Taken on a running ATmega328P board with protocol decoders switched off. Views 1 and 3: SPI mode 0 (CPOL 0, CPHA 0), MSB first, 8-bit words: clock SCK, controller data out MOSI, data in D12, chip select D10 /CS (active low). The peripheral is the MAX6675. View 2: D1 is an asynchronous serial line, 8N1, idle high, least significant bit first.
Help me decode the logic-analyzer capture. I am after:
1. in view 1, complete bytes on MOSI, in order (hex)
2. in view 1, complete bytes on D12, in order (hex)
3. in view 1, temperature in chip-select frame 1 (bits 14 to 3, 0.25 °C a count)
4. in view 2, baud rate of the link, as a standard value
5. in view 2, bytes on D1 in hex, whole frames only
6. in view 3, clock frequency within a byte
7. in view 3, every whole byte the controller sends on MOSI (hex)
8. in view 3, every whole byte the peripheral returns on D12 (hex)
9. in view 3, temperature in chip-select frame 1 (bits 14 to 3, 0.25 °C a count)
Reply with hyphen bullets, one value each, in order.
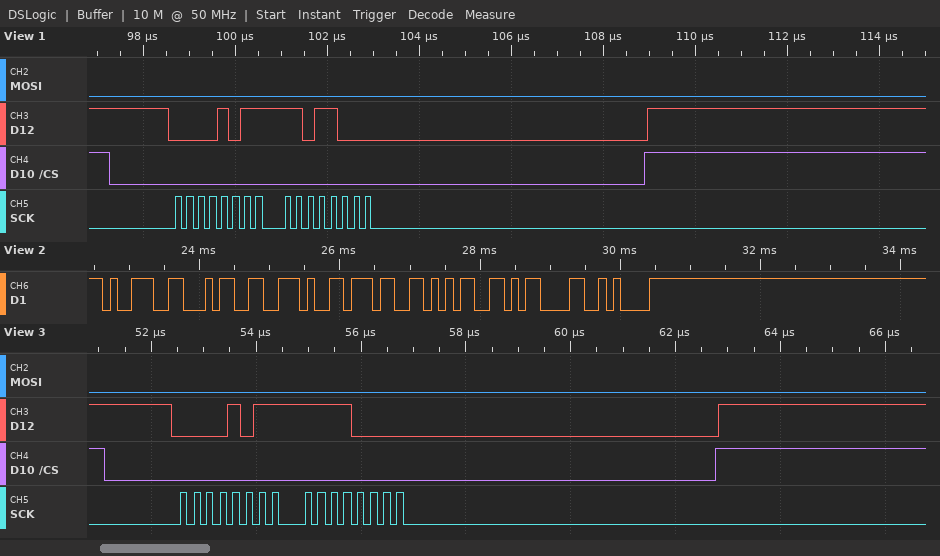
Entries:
- 0x00 0x00
- 0x0B 0xD8
- 94.75 °C
- 9600 baud
- 39 34 2E 37 35 0D 0A
- 4 MHz
- 00 00
- 0B F0
- 95.50 °C
